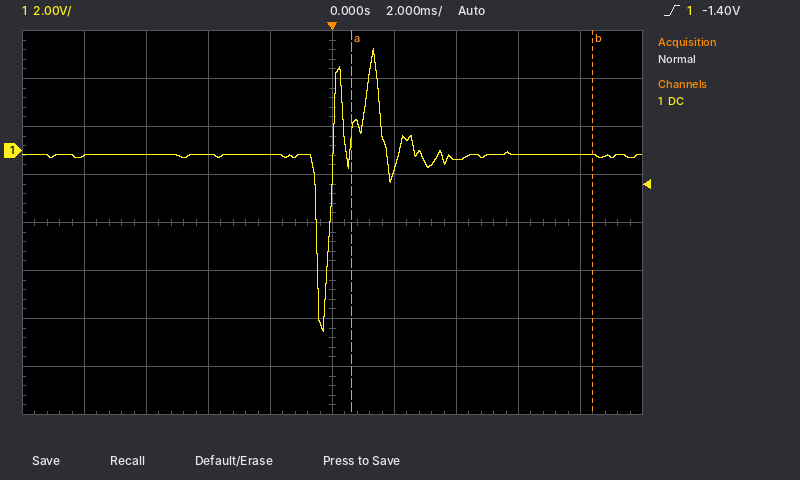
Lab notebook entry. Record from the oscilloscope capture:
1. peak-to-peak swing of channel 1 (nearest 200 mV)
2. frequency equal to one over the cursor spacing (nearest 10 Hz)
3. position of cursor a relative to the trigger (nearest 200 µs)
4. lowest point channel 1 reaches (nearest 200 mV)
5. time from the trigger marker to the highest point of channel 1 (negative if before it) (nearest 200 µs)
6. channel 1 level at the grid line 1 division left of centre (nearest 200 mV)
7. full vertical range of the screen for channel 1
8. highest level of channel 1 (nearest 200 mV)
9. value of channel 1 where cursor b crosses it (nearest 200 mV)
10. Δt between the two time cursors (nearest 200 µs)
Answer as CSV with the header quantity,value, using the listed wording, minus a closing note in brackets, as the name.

quantity,value
peak-to-peak swing of channel 1,11.8 V
frequency equal to one over the cursor spacing,130 Hz
position of cursor a relative to the trigger,+600 µs
lowest point channel 1 reaches,-7.6 V
time from the trigger marker to the highest point of channel 1 (negative if before it),+1.4 ms
channel 1 level at the grid line 1 division left of centre,-200 mV
full vertical range of the screen for channel 1,16 V
highest level of channel 1,4.2 V
value of channel 1 where cursor b crosses it,-200 mV
Δt between the two time cursors,7.8 ms
